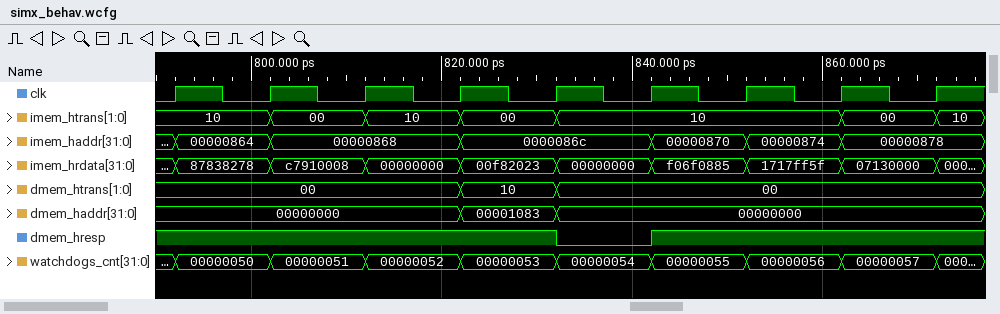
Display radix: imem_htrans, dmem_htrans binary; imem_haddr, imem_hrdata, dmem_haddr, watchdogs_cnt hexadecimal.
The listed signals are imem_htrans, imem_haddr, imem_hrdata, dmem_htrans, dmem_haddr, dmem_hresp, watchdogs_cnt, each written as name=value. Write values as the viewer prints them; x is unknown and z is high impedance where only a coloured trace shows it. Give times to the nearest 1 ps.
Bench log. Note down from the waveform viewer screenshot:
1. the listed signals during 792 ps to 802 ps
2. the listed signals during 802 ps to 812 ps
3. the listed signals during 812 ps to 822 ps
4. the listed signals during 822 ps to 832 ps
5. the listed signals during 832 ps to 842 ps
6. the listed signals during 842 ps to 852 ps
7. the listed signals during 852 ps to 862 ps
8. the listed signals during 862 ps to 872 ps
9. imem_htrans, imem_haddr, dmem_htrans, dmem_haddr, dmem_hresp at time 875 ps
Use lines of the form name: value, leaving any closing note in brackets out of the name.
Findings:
the listed signals during 792 ps to 802 ps: imem_htrans=10, imem_haddr=00000864, imem_hrdata=87838278, dmem_htrans=00, dmem_haddr=00000000, dmem_hresp=1, watchdogs_cnt=00000050
the listed signals during 802 ps to 812 ps: imem_htrans=00, imem_haddr=00000868, imem_hrdata=c7910008, dmem_htrans=00, dmem_haddr=00000000, dmem_hresp=1, watchdogs_cnt=00000051
the listed signals during 812 ps to 822 ps: imem_htrans=10, imem_haddr=00000868, imem_hrdata=00000000, dmem_htrans=00, dmem_haddr=00000000, dmem_hresp=1, watchdogs_cnt=00000052
the listed signals during 822 ps to 832 ps: imem_htrans=00, imem_haddr=0000086c, imem_hrdata=00f82023, dmem_htrans=10, dmem_haddr=00001083, dmem_hresp=1, watchdogs_cnt=00000053
the listed signals during 832 ps to 842 ps: imem_htrans=10, imem_haddr=0000086c, imem_hrdata=00000000, dmem_htrans=00, dmem_haddr=00000000, dmem_hresp=0, watchdogs_cnt=00000054
the listed signals during 842 ps to 852 ps: imem_htrans=10, imem_haddr=00000870, imem_hrdata=f06f0885, dmem_htrans=00, dmem_haddr=00000000, dmem_hresp=1, watchdogs_cnt=00000055
the listed signals during 852 ps to 862 ps: imem_htrans=10, imem_haddr=00000874, imem_hrdata=1717ff5f, dmem_htrans=00, dmem_haddr=00000000, dmem_hresp=1, watchdogs_cnt=00000056
the listed signals during 862 ps to 872 ps: imem_htrans=00, imem_haddr=00000878, imem_hrdata=07130000, dmem_htrans=00, dmem_haddr=00000000, dmem_hresp=1, watchdogs_cnt=00000057
imem_htrans, imem_haddr, dmem_htrans, dmem_haddr, dmem_hresp at time 875 ps: imem_htrans=10, imem_haddr=00000878, dmem_htrans=00, dmem_haddr=00000000, dmem_hresp=1
